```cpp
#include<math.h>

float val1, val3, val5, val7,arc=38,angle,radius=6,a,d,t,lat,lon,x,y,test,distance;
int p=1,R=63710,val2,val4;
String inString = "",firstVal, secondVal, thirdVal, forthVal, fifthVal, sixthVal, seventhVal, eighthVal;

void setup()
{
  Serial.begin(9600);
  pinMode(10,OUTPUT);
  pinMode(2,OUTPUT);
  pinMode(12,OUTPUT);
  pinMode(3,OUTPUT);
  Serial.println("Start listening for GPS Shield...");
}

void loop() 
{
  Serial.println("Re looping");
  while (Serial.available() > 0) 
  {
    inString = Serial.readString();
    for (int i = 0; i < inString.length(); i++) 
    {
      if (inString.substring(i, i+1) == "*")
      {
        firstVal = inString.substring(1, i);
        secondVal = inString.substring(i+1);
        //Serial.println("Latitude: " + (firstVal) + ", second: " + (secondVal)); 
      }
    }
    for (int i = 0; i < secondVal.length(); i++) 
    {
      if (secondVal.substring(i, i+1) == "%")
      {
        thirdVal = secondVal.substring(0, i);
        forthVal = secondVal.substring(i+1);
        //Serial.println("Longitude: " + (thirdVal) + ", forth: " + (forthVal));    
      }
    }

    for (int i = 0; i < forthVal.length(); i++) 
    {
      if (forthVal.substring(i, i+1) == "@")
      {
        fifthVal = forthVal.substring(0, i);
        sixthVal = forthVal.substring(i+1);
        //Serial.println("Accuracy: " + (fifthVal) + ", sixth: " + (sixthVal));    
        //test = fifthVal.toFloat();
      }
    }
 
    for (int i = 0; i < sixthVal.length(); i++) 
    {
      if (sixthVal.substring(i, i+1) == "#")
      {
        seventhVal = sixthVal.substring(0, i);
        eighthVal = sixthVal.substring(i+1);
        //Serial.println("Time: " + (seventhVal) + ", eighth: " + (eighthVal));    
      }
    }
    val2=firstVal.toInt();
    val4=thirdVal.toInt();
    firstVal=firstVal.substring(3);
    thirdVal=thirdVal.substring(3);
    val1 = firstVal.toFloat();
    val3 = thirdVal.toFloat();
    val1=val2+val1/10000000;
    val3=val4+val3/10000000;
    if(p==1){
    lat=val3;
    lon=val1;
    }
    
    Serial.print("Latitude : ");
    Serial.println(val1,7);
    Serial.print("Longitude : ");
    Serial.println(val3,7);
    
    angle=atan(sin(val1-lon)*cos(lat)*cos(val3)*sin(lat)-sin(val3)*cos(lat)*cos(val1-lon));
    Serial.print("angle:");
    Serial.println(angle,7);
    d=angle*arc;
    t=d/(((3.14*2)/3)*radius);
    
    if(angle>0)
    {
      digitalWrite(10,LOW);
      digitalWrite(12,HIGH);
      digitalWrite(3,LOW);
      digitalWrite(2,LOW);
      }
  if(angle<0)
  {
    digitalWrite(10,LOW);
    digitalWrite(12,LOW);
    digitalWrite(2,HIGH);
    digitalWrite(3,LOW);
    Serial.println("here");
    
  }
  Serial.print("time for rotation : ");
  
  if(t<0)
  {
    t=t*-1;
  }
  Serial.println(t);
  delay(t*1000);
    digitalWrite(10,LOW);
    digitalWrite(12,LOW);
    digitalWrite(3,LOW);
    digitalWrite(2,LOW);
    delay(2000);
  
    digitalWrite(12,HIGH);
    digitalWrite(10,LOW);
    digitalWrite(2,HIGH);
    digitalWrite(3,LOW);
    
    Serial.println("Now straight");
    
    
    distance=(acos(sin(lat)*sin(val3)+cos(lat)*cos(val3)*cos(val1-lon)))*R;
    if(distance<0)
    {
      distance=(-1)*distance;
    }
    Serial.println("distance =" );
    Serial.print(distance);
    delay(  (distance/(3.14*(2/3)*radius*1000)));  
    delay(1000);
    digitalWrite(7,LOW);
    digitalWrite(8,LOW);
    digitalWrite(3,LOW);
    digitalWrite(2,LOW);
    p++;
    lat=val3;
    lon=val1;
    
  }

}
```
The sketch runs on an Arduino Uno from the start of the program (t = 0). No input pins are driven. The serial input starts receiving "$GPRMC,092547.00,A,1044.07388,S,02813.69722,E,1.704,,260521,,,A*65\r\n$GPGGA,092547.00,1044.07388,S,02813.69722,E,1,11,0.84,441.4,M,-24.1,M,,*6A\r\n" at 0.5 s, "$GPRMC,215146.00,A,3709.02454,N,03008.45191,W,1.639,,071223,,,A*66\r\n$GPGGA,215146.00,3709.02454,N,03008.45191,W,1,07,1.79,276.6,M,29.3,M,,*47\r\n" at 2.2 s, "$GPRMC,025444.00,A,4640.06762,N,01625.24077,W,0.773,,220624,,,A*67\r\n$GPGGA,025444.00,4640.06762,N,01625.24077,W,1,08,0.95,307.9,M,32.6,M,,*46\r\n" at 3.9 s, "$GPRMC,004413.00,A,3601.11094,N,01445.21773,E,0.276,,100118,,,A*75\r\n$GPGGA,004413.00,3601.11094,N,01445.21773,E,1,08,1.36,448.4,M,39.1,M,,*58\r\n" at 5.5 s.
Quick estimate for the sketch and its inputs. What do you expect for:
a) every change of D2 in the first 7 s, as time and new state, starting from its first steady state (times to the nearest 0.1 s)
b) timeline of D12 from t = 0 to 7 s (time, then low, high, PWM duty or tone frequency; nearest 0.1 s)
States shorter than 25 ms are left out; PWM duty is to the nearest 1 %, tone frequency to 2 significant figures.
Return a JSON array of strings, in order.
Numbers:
["0 s low; 3.7 s high; 4.7 s low", "0 s low; 3.7 s high; 6.7 s low"]
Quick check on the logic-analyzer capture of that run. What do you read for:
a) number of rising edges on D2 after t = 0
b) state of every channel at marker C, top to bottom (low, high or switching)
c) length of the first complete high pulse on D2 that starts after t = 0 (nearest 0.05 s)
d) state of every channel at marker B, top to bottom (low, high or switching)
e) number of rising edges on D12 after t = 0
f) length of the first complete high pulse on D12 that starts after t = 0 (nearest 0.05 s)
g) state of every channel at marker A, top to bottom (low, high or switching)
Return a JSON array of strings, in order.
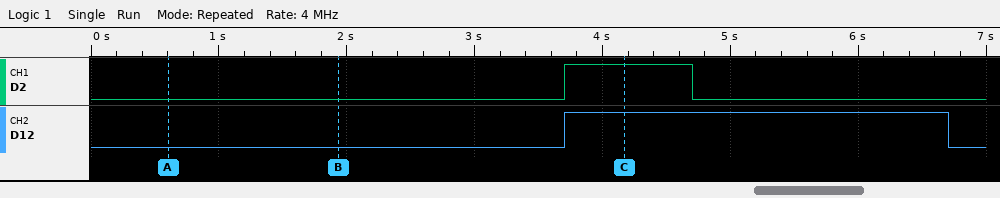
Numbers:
["1", "D2 high, D12 high", "1.00 s", "D2 low, D12 low", "1", "3.00 s", "D2 low, D12 low"]
